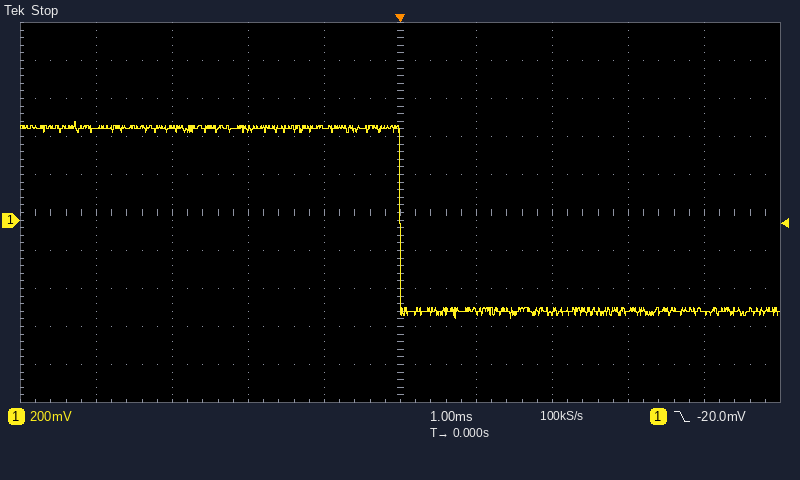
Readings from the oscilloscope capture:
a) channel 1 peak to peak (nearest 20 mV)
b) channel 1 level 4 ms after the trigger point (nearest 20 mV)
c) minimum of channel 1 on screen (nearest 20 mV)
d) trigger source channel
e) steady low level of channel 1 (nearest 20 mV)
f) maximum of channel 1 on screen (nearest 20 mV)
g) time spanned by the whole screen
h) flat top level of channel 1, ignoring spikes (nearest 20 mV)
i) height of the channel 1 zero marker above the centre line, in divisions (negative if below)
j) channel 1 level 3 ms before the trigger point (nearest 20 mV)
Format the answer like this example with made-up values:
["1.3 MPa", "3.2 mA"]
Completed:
["1.04 V", "-480 mV", "-520 mV", "channel 1", "-480 mV", "520 mV", "10 ms", "480 mV", "-0.2 div", "480 mV"]
